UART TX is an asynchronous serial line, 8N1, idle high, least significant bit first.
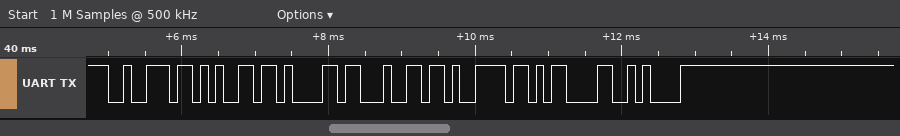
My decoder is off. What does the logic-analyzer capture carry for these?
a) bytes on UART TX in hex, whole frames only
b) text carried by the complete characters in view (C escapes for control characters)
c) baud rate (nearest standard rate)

0x72 0x65 0x61 0x64 0x79 0x0D 0x0A
"ready\r\n"
9600 baud
